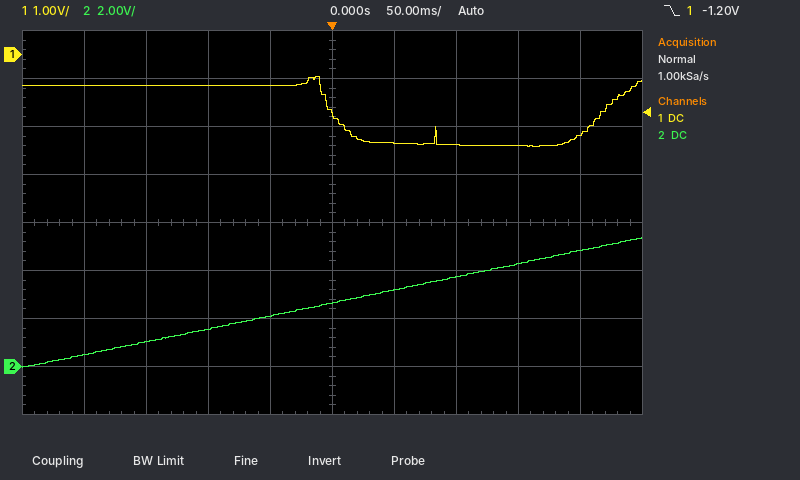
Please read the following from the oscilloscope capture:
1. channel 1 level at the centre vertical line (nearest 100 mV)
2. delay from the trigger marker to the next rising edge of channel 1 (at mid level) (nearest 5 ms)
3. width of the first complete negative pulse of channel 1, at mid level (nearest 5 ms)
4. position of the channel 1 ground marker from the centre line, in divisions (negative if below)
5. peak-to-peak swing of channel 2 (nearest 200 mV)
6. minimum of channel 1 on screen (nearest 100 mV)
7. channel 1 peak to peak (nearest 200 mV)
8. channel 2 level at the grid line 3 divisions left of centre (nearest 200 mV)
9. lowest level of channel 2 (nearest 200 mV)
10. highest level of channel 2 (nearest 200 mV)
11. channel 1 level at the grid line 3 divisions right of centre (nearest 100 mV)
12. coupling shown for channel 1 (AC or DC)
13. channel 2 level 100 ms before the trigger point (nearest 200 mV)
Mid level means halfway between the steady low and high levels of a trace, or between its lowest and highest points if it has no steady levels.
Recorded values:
-1.2 V
215 ms
215 ms
+3.5 div
5.4 V
-1.9 V
1.4 V
1.0 V
0.0 V
5.4 V
-1.9 V
DC
1.6 V
